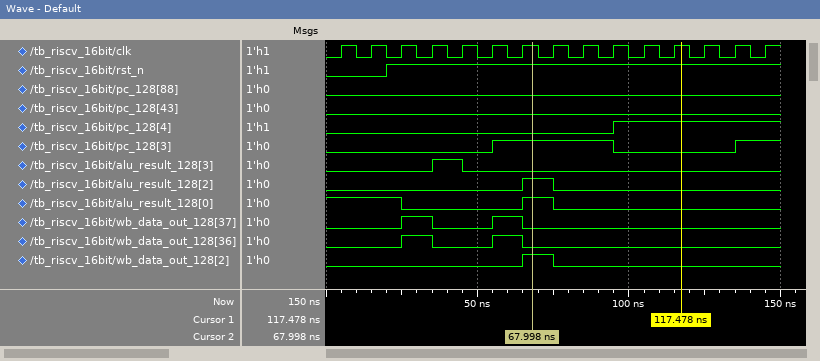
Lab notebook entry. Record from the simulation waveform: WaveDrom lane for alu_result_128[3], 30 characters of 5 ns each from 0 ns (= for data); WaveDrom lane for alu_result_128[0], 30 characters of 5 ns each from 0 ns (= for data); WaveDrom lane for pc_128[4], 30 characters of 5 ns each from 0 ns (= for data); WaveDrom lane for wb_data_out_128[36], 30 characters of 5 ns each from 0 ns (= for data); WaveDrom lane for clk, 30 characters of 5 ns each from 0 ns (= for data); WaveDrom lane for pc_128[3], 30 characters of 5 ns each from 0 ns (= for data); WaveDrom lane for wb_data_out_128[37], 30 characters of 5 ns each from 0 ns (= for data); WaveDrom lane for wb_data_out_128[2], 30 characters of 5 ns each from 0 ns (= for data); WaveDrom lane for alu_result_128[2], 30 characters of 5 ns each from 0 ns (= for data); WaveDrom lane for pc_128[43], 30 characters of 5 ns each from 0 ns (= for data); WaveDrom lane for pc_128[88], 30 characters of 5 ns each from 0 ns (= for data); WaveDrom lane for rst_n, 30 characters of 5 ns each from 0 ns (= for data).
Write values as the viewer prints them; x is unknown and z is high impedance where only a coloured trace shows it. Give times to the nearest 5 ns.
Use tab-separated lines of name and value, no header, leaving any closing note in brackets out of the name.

WaveDrom lane for alu_result_128[3], 30 characters of 5 ns each from 0 ns	{name: 'alu_result_128[3]', wave: '0......1.0....................'}
WaveDrom lane for alu_result_128[0], 30 characters of 5 ns each from 0 ns	{name: 'alu_result_128[0]', wave: '1....0.......1.0..............'}
WaveDrom lane for pc_128[4], 30 characters of 5 ns each from 0 ns	{name: 'pc_128[4]', wave: '0..................1..........'}
WaveDrom lane for wb_data_out_128[36], 30 characters of 5 ns each from 0 ns	{name: 'wb_data_out_128[36]', wave: '0....1.0...1.0................'}
WaveDrom lane for clk, 30 characters of 5 ns each from 0 ns	{name: 'clk', wave: '010101010101010101010101010101'}
WaveDrom lane for pc_128[3], 30 characters of 5 ns each from 0 ns	{name: 'pc_128[3]', wave: '0..........1.......0.......1..'}
WaveDrom lane for wb_data_out_128[37], 30 characters of 5 ns each from 0 ns	{name: 'wb_data_out_128[37]', wave: '0....1.0...1.0................'}
WaveDrom lane for wb_data_out_128[2], 30 characters of 5 ns each from 0 ns	{name: 'wb_data_out_128[2]', wave: '0............1.0..............'}
WaveDrom lane for alu_result_128[2], 30 characters of 5 ns each from 0 ns	{name: 'alu_result_128[2]', wave: '0............1.0..............'}
WaveDrom lane for pc_128[43], 30 characters of 5 ns each from 0 ns	{name: 'pc_128[43]', wave: '0.............................'}
WaveDrom lane for pc_128[88], 30 characters of 5 ns each from 0 ns	{name: 'pc_128[88]', wave: '0.............................'}
WaveDrom lane for rst_n, 30 characters of 5 ns each from 0 ns	{name: 'rst_n', wave: '0...1.........................'}
